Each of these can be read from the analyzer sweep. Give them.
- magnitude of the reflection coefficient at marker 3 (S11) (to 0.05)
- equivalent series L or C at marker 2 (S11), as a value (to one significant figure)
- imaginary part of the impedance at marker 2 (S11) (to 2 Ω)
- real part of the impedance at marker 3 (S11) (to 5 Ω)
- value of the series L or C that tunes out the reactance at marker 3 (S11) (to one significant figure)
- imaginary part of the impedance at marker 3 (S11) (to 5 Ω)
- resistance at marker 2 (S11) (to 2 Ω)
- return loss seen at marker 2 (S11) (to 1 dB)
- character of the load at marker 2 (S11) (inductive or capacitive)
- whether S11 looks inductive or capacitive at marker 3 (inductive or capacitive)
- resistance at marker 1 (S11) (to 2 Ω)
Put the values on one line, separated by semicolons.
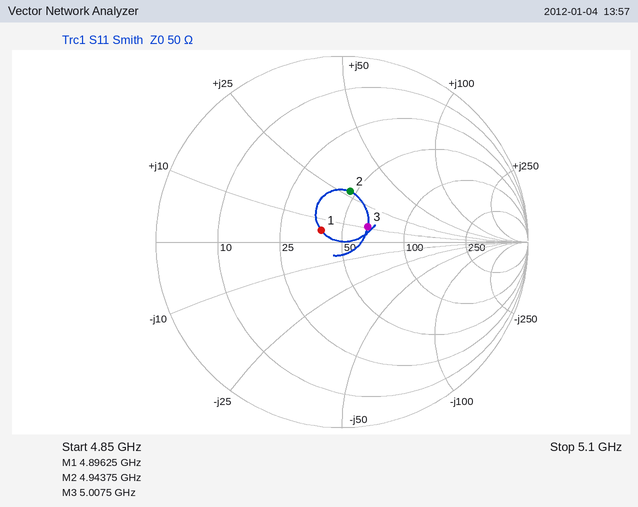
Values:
0.15; 900 pH; +28 Ω; 65 Ω; 3 pF; +10 Ω; 46 Ω; 11 dB; inductive; inductive; 40 Ω
